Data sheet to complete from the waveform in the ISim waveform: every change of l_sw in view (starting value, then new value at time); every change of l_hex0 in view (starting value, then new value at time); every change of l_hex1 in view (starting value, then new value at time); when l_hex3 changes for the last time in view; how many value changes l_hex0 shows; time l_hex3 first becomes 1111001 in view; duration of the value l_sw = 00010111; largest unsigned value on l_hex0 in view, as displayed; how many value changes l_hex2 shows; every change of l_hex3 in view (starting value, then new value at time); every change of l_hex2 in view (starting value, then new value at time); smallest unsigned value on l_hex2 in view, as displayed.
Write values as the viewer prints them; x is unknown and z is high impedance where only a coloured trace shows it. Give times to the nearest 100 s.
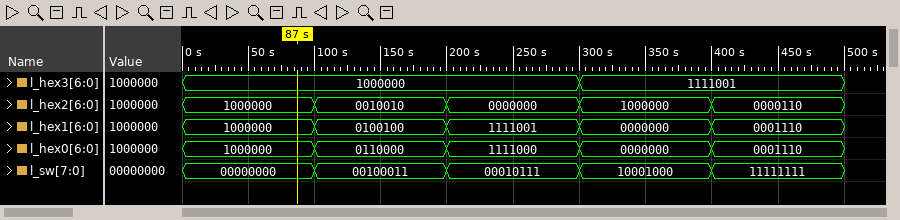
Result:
00000000, 00100011 at 100 s, 00010111 at 200 s, 10001000 at 300 s, 11111111 at 400 s
1000000, 0110000 at 100 s, 1111000 at 200 s, 0000000 at 300 s, 0001110 at 400 s
1000000, 0100100 at 100 s, 1111001 at 200 s, 0000000 at 300 s, 0001110 at 400 s
300 s
4
300 s
100 s
1111000
4
1000000, 1111001 at 300 s
1000000, 0010010 at 100 s, 0000000 at 200 s, 1000000 at 300 s, 0000110 at 400 s
0000000
